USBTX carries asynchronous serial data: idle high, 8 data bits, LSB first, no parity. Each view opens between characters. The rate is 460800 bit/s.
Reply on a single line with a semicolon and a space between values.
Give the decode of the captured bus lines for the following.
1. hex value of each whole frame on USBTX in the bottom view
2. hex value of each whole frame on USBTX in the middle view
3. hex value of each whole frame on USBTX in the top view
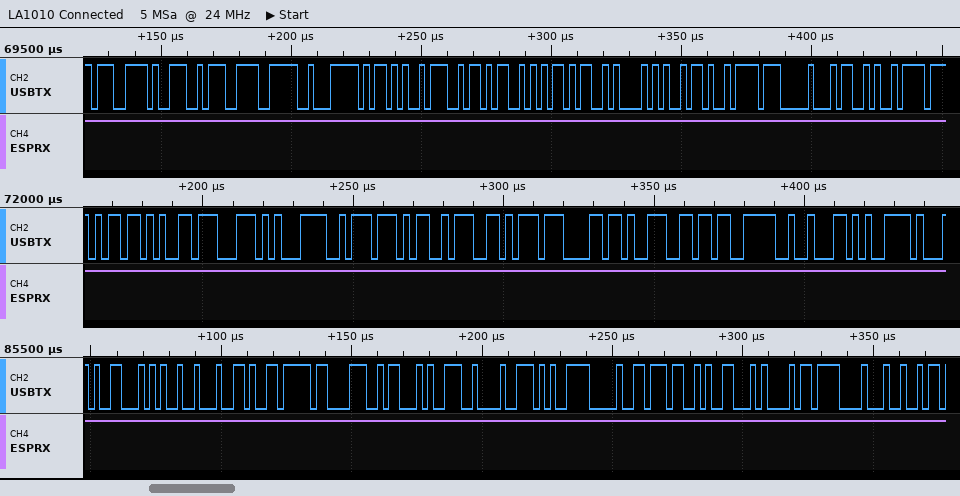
19, 25, 64, F6, C3, 1A, 39, C8, E5, 90, 37, 19, A1, 0F, 24; 6D, D9, 5C, 3C, 77, D3, D6, 87, CB, B6, 3E, 62, 79; E7, 39, E7, 3E, 7C, 2B, A7, 4D, AD, 0A, A5, E9, 07, 34, E9
